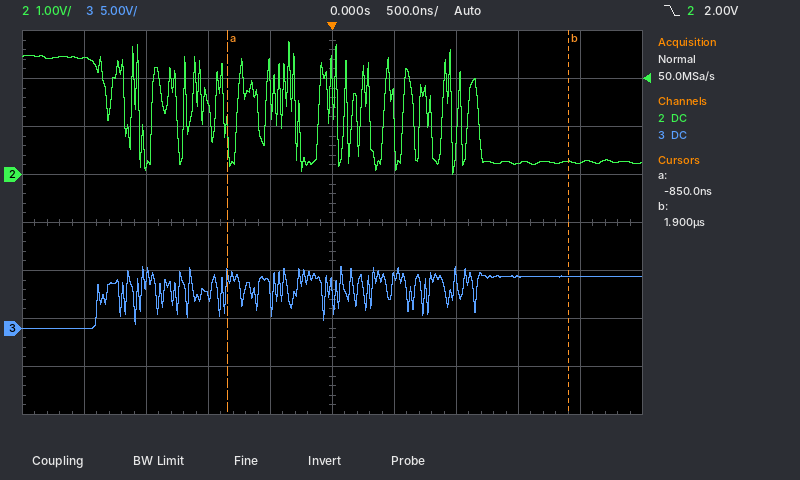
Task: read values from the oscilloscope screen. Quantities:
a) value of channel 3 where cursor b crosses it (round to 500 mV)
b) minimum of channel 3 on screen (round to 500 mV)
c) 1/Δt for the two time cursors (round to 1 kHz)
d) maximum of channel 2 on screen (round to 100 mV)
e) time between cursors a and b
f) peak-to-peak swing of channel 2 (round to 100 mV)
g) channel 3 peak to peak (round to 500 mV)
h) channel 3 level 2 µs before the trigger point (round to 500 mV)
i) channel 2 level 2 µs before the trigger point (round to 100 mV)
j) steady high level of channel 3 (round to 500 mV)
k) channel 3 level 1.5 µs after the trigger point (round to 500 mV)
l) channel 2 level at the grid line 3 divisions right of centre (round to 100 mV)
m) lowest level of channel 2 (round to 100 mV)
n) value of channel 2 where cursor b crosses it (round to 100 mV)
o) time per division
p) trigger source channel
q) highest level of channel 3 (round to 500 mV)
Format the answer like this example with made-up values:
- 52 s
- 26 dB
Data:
- 5.5 V
- 0.0 V
- 364 kHz
- 2.8 V
- 2.75 µs
- 2.8 V
- 6.5 V
- 0.0 V
- 2.4 V
- 5.5 V
- 5.5 V
- 200 mV
- 0.0 V
- 300 mV
- 500 ns
- channel 2
- 6.5 V
